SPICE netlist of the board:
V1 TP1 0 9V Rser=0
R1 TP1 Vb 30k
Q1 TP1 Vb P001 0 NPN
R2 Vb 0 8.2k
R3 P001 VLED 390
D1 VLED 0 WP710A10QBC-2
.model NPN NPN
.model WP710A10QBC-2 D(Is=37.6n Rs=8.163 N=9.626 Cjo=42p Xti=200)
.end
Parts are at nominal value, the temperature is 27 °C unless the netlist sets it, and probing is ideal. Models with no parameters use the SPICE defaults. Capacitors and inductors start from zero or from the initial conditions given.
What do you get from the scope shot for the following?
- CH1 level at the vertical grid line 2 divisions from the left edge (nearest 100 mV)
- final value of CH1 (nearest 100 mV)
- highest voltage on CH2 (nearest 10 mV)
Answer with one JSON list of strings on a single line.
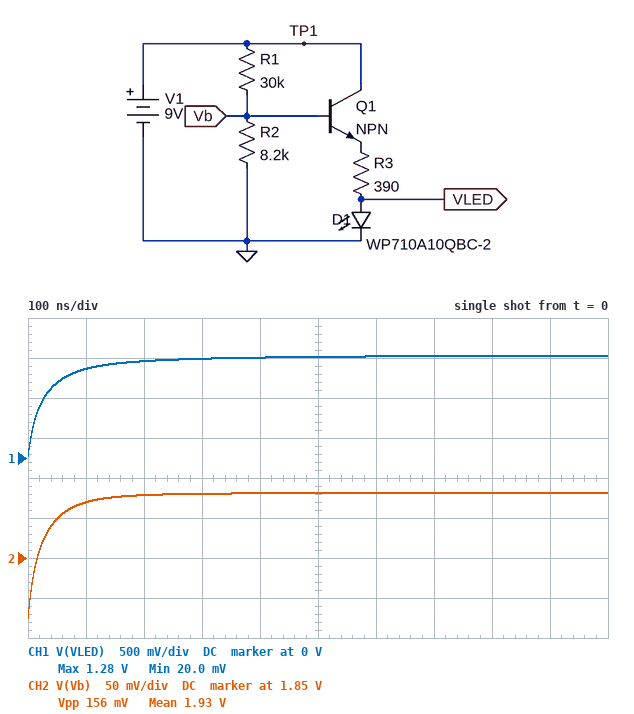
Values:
["1.2 V", "1.3 V", "1.93 V"]
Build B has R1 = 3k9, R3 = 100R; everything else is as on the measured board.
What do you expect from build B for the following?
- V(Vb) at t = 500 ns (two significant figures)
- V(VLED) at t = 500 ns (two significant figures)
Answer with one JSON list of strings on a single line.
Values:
["5.7 V", "3.3 V"]
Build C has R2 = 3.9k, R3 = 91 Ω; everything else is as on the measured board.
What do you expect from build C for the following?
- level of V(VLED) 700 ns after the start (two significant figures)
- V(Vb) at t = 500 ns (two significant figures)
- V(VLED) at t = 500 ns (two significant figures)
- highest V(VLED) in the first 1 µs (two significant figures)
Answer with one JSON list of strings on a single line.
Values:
["420 mV", "1.0 V", "410 mV", "430 mV"]
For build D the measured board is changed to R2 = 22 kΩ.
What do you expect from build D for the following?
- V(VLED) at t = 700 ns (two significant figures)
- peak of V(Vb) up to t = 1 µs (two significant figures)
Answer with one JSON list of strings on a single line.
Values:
["2.5 V", "3.7 V"]
